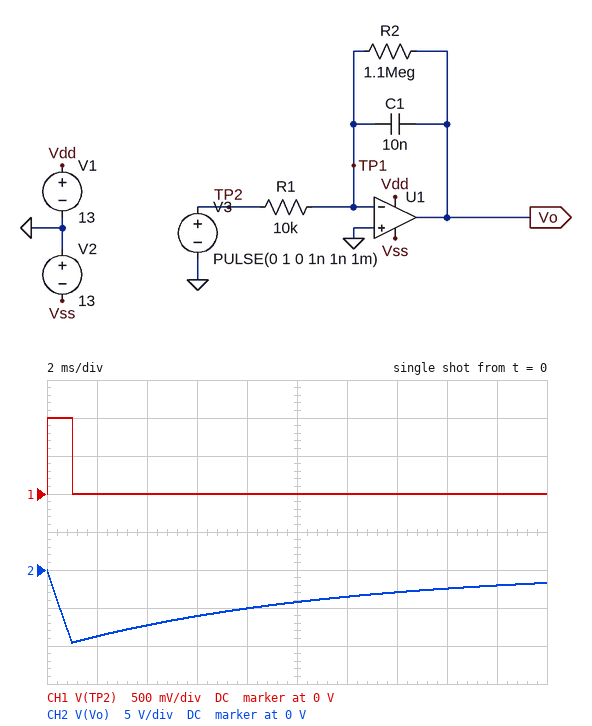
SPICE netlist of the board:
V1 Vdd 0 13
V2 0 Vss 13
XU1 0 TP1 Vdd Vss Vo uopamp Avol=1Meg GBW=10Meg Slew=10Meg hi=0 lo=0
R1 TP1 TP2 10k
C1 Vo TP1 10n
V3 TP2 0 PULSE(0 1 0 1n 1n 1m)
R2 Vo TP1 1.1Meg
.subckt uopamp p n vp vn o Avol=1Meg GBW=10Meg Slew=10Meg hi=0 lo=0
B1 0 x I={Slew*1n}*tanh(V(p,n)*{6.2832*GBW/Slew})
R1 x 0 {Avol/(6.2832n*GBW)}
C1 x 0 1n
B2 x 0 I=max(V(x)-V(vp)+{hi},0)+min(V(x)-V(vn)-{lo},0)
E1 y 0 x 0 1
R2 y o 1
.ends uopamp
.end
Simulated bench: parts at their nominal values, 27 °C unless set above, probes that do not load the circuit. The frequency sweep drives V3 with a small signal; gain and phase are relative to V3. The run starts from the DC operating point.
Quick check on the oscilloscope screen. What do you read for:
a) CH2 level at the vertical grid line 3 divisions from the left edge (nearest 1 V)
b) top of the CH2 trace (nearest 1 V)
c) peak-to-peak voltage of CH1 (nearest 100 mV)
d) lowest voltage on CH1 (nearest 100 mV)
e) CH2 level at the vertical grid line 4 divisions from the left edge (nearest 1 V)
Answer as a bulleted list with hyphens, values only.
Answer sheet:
- -6 V
- 0 V
- 1.0 V
- 0 V
- -5 V
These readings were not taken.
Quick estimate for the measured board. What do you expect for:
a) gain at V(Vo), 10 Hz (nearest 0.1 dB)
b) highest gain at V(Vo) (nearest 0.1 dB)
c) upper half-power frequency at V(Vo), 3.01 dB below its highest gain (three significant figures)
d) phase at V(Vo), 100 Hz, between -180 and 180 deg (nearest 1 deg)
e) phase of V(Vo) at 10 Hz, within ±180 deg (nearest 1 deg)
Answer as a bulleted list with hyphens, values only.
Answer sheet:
- 39.1 dB
- 40.8 dB
- 14.5 Hz
- 98 deg
- 145 deg
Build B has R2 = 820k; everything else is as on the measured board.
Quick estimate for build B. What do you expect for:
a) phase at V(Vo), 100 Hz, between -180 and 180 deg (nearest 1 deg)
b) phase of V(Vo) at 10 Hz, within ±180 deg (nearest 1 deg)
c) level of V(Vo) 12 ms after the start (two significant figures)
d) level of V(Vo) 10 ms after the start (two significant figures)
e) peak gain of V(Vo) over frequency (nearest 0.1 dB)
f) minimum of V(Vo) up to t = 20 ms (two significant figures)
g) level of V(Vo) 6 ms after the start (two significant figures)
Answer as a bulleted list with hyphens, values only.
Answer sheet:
- 101 deg
- 153 deg
- -2.5 V
- -3.1 V
- 38.3 dB
- -9.4 V
- -5.1 V
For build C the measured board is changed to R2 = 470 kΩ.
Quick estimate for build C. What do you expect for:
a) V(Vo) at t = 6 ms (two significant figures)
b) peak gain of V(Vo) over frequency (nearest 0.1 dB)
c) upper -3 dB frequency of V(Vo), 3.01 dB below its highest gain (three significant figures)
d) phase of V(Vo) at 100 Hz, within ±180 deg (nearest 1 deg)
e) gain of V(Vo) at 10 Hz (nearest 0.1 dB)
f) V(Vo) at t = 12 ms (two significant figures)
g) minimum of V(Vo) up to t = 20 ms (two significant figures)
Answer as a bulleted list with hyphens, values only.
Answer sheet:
- -3.1 V
- 33.4 dB
- 33.9 Hz
- 109 deg
- 33.1 dB
- -870 mV
- -9.0 V
